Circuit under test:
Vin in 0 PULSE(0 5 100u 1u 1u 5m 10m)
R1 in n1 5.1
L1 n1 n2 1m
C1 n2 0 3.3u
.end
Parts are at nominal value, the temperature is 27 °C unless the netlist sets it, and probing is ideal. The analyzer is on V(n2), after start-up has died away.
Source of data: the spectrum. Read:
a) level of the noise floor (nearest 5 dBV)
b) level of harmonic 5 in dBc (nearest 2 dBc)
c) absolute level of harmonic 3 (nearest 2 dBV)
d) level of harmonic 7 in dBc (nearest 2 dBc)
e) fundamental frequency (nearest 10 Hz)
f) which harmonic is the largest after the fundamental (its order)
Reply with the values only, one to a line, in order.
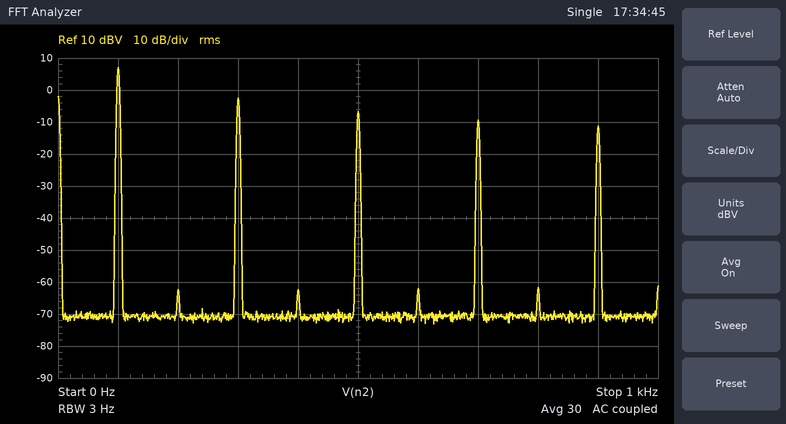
-70 dBV
-14 dBc
-2 dBV
-16 dBc
100 Hz
3
